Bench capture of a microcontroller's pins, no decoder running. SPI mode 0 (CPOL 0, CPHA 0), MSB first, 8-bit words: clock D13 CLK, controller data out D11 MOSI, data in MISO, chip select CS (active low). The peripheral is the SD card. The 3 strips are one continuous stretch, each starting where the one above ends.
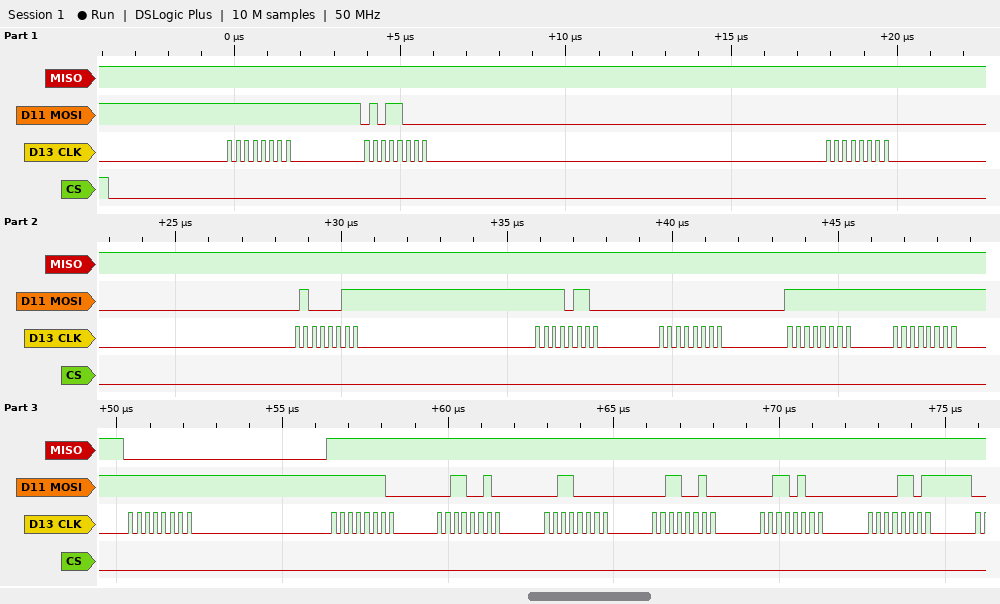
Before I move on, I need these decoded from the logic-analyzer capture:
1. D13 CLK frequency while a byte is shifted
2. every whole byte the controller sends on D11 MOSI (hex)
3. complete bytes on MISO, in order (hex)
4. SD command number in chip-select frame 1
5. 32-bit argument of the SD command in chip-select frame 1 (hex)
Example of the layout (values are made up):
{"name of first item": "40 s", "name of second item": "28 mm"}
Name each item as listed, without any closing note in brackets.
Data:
{"D13 CLK frequency while a byte is shifted": "4 MHz", "every whole byte the controller sends on D11 MOSI": "0xFF 0x58 0x00 0x43 0xF6 0x00 0xFF 0xFF 0xFF 0xFE 0x32 0x30 0x32 0x34 0x0D", "complete bytes on MISO, in order": "0xFF 0xFF 0xFF 0xFF 0xFF 0xFF 0xFF 0xFF 0x00 0xFF 0xFF 0xFF 0xFF 0xFF 0xFF", "SD command number in chip-select frame 1": "CMD24", "32-bit argument of the SD command in chip-select frame 1": "0x0043F600"}
